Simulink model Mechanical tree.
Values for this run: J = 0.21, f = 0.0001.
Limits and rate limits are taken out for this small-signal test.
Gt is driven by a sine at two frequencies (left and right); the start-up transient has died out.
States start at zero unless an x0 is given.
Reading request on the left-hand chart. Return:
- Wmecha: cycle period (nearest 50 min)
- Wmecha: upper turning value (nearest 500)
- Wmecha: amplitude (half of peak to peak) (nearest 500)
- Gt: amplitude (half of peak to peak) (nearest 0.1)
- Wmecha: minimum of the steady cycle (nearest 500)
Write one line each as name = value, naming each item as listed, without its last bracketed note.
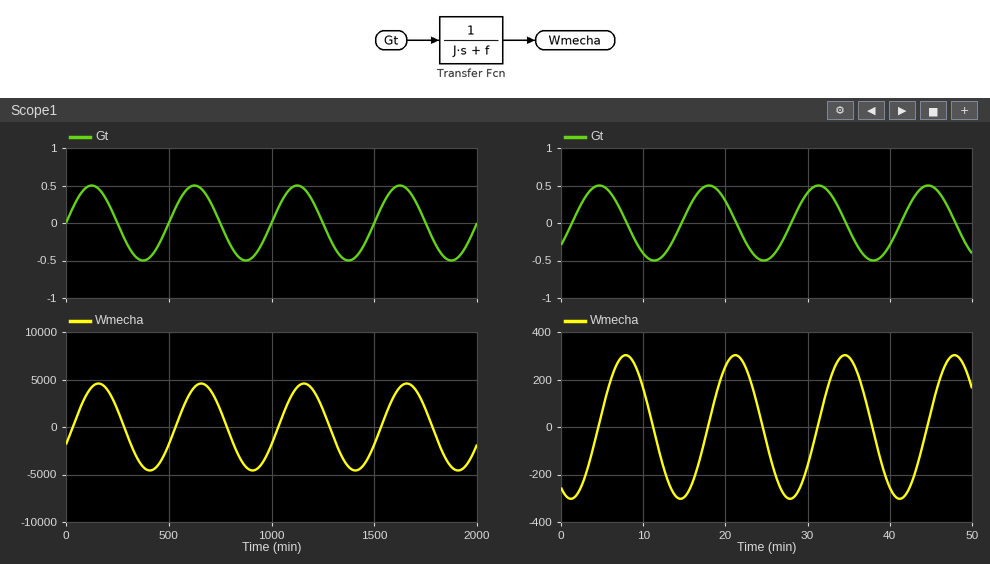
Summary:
Wmecha: cycle period = 500 min
Wmecha: upper turning value = 4500
Wmecha: amplitude (half of peak to peak) = 4500
Gt: amplitude (half of peak to peak) = 0.5
Wmecha: minimum of the steady cycle = -4500
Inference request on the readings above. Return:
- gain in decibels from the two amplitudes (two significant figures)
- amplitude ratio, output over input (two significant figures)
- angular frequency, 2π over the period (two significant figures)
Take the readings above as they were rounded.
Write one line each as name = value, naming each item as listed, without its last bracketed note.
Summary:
gain in decibels from the two amplitudes = 79 dB
amplitude ratio, output over input = 9000
angular frequency, 2π over the period = 0.013 rad/min
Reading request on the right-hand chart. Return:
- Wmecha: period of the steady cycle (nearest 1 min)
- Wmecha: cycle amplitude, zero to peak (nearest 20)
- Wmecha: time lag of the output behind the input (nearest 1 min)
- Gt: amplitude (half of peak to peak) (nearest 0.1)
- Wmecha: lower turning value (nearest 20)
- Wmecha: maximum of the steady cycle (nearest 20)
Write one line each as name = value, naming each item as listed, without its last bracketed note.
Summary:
Wmecha: period of the steady cycle = 13 min
Wmecha: cycle amplitude, zero to peak = 300
Wmecha: time lag of the output behind the input = 3 min
Gt: amplitude (half of peak to peak) = 0.5
Wmecha: lower turning value = -300
Wmecha: maximum of the steady cycle = 300
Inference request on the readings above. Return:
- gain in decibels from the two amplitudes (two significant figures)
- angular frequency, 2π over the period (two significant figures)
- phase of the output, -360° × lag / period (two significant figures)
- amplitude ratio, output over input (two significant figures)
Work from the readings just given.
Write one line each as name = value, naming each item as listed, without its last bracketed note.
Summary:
gain in decibels from the two amplitudes = 56 dB
angular frequency, 2π over the period = 0.48 rad/min
phase of the output, -360° × lag / period = -83°
amplitude ratio, output over input = 600
